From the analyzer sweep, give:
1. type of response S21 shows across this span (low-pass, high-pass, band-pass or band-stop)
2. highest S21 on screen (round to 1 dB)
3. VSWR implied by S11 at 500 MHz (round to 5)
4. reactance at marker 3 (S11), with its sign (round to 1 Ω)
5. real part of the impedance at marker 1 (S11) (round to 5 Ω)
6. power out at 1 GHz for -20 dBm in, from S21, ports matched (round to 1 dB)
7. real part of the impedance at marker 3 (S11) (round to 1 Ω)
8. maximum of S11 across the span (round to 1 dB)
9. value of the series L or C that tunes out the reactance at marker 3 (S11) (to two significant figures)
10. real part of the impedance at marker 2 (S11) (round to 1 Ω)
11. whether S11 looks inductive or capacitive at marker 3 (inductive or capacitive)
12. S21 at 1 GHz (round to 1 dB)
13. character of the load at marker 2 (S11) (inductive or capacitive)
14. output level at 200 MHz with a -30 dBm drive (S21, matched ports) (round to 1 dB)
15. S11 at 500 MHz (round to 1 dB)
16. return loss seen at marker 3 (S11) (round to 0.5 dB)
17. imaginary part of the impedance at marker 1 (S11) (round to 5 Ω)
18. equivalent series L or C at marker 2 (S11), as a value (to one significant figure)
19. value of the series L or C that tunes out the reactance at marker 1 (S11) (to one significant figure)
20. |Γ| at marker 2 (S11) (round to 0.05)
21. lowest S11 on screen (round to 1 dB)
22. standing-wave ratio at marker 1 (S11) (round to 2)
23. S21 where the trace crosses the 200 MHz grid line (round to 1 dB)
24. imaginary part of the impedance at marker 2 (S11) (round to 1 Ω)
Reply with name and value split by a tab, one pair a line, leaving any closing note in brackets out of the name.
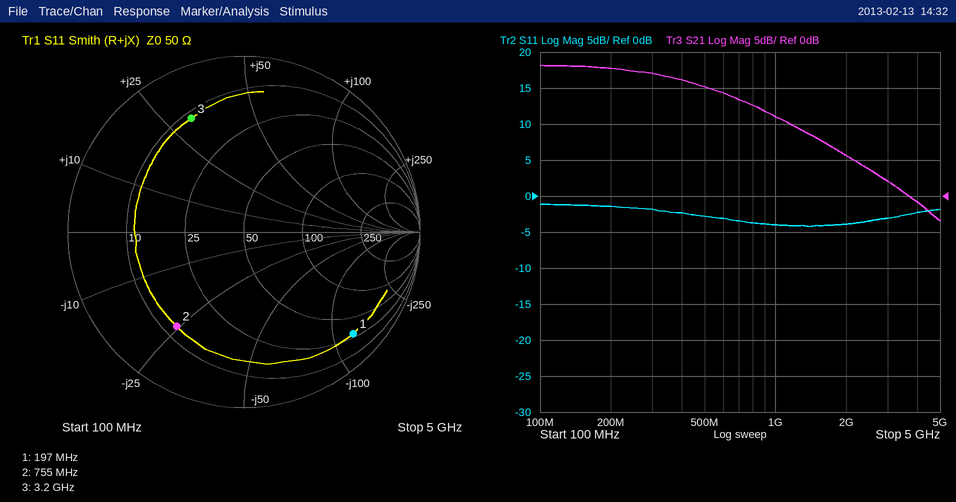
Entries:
type of response S21 shows across this span	low-pass
highest S21 on screen	18 dB
VSWR implied by S11 at 500 MHz	5
reactance at marker 3 (S11), with its sign	+31 Ω
real part of the impedance at marker 1 (S11)	30 Ω
power out at 1 GHz for -20 dBm in, from S21, ports matched	-9 dBm
real part of the impedance at marker 3 (S11)	12 Ω
maximum of S11 across the span	-1 dB
value of the series L or C that tunes out the reactance at marker 3 (S11)	1.6 pF
real part of the impedance at marker 2 (S11)	13 Ω
whether S11 looks inductive or capacitive at marker 3	inductive
S21 at 1 GHz	11 dB
character of the load at marker 2 (S11)	capacitive
output level at 200 MHz with a -30 dBm drive (S21, matched ports)	-12 dBm
S11 at 500 MHz	-3 dB
return loss seen at marker 3 (S11)	3.0 dB
imaginary part of the impedance at marker 1 (S11)	-120 Ω
equivalent series L or C at marker 2 (S11), as a value	9 pF
value of the series L or C that tunes out the reactance at marker 1 (S11)	100 nH
|Γ| at marker 2 (S11)	0.65
lowest S11 on screen	-4 dB
standing-wave ratio at marker 1 (S11)	12
S21 where the trace crosses the 200 MHz grid line	18 dB
imaginary part of the impedance at marker 2 (S11)	-24 Ω
